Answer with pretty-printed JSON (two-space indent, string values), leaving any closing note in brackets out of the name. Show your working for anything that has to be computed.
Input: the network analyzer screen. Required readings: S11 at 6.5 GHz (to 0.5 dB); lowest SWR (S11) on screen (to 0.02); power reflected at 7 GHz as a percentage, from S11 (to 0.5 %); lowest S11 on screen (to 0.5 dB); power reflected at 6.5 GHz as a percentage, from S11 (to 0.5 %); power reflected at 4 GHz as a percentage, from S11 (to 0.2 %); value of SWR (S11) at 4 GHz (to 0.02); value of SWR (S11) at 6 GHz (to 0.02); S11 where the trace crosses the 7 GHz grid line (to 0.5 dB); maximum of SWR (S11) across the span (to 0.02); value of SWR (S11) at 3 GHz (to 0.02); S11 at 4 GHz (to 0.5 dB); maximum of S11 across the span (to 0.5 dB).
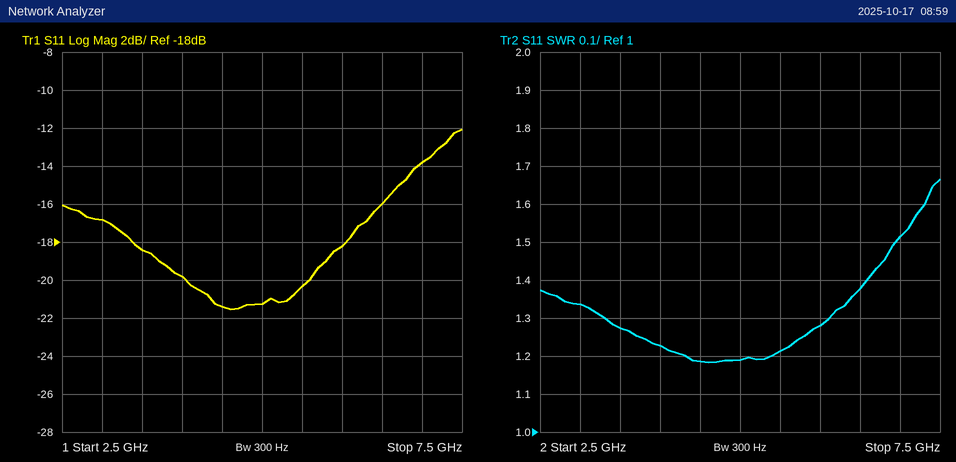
{
  "S11 at 6.5 GHz": "-16.0 dB",
  "lowest SWR (S11) on screen": "1.18",
  "power reflected at 7 GHz as a percentage, from S11": "10^(-14/10) ≈ 4.0 %",
  "lowest S11 on screen": "-21.5 dB",
  "power reflected at 6.5 GHz as a percentage, from S11": "10^(-16/10) ≈ 2.5 %",
  "power reflected at 4 GHz as a percentage, from S11": "10^(-20/10) ≈ 1.0 %",
  "value of SWR (S11) at 4 GHz": "1.22",
  "value of SWR (S11) at 6 GHz": "1.28",
  "S11 where the trace crosses the 7 GHz grid line": "-14.0 dB",
  "maximum of SWR (S11) across the span": "1.66",
  "value of SWR (S11) at 3 GHz": "1.34",
  "S11 at 4 GHz": "-20.0 dB",
  "maximum of S11 across the span": "-12.0 dB"
}
